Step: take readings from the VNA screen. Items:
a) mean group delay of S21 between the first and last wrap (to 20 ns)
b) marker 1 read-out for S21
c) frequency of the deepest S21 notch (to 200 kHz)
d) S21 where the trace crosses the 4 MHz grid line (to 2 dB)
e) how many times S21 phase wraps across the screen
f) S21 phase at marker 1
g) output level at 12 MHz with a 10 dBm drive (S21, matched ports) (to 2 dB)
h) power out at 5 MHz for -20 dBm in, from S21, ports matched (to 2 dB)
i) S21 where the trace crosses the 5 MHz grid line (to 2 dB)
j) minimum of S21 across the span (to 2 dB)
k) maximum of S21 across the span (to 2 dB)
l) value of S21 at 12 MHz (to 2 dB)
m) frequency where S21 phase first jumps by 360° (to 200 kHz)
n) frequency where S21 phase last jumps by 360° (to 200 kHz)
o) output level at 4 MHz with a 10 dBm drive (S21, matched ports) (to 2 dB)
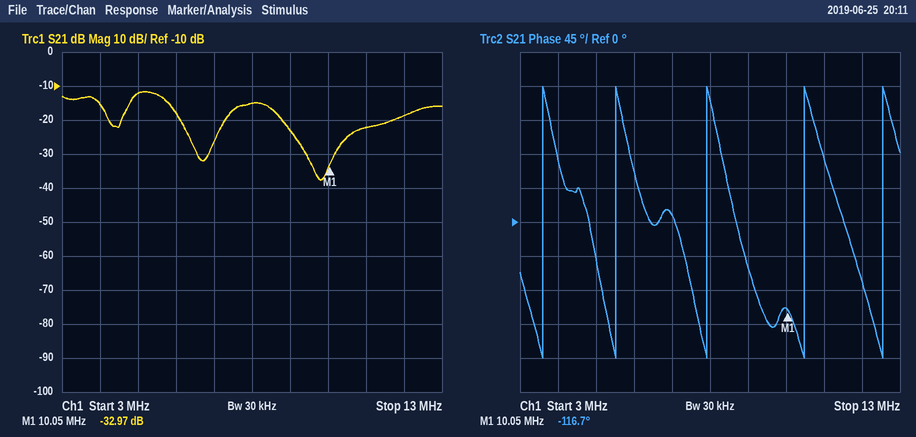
440 ns
-32.97 dB
9.8 MHz
-16 dB
5
-116.7°
-8 dBm
-32 dBm
-12 dB
-38 dB
-12 dB
-18 dB
3.6 MHz
12.6 MHz
-6 dBm
